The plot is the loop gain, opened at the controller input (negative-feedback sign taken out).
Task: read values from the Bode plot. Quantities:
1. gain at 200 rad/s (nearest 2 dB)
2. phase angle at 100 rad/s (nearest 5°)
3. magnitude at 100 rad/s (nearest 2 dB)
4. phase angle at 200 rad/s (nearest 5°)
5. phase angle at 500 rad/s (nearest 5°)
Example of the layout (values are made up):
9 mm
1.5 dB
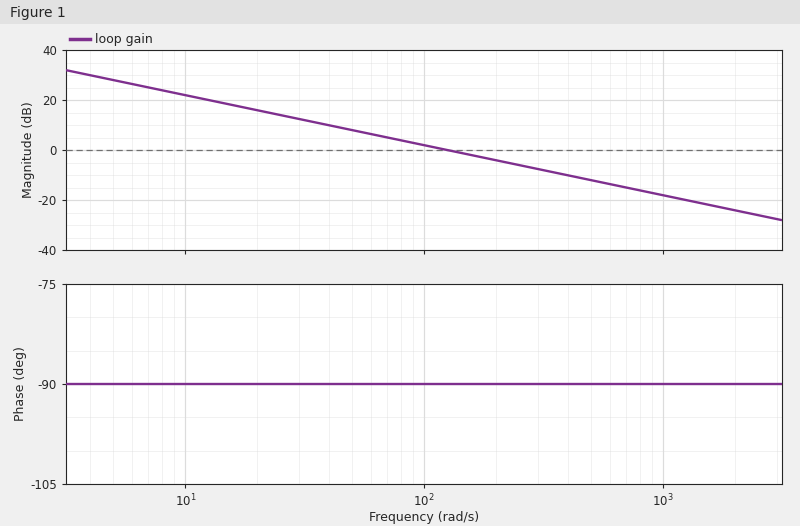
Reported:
-4 dB
-90°
2 dB
-90°
-90°
